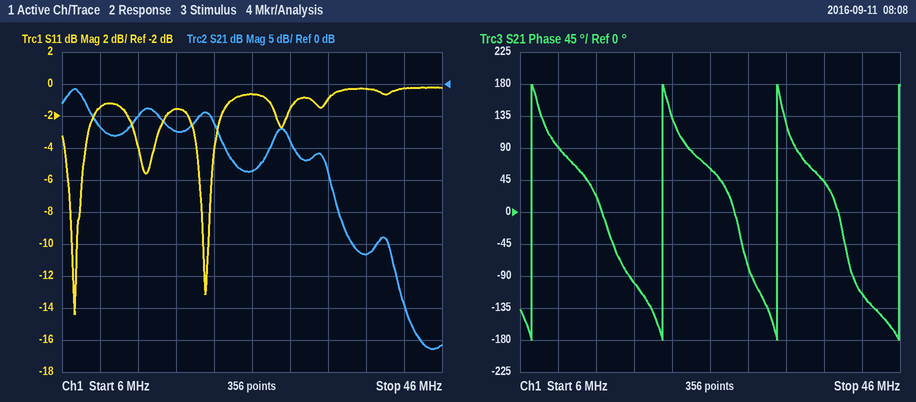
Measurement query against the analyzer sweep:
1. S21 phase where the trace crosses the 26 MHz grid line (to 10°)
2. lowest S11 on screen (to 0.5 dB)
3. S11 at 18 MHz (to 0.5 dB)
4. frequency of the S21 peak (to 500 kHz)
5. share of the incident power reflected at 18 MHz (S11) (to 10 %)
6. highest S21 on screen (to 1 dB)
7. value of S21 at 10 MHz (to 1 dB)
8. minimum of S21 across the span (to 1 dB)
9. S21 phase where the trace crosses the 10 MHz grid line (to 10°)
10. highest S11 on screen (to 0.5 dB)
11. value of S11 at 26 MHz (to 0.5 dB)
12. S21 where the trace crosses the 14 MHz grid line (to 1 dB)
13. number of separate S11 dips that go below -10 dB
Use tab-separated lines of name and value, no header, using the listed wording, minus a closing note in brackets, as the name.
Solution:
S21 phase where the trace crosses the 26 MHz grid line	60°
lowest S11 on screen	-14.5 dB
S11 at 18 MHz	-1.5 dB
frequency of the S21 peak	7.5 MHz
share of the incident power reflected at 18 MHz (S11)	70 %
highest S21 on screen	-1 dB
value of S21 at 10 MHz	-7 dB
minimum of S21 across the span	-41 dB
S21 phase where the trace crosses the 10 MHz grid line	90°
highest S11 on screen	0.0 dB
value of S11 at 26 MHz	-0.5 dB
S21 where the trace crosses the 14 MHz grid line	-5 dB
number of separate S11 dips that go below -10 dB	2
